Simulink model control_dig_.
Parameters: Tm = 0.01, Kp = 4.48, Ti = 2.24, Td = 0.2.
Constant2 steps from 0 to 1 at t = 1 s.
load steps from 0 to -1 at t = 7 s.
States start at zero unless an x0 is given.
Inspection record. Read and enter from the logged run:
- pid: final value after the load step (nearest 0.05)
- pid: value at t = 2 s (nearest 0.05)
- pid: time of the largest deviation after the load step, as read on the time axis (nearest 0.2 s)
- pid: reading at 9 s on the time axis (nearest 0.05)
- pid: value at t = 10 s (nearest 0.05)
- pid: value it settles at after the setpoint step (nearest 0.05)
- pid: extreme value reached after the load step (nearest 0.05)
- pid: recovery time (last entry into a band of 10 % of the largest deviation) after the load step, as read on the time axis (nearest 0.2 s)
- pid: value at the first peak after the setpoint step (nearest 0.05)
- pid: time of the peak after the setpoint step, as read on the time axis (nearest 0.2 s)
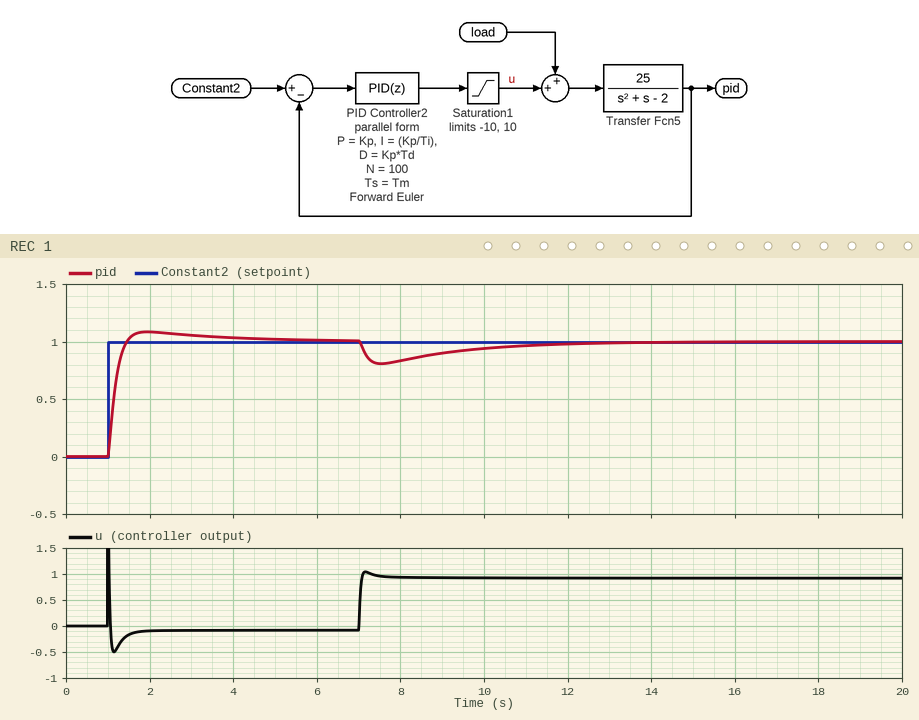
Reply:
1.00
1.10
7.6 s
0.90
0.95
1.00
0.80
12.2 s
1.10
2.0 s
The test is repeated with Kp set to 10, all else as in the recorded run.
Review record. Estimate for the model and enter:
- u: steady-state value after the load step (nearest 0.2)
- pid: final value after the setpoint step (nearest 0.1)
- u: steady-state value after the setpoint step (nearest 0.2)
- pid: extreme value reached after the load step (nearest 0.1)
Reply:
1.0
1.0
0.0
0.9
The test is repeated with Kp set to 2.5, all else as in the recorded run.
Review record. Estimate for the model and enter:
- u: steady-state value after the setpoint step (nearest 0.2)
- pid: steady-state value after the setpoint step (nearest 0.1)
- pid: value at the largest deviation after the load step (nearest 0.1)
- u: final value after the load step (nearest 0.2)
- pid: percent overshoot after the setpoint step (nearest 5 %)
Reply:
0.0
1.0
0.6
1.0
10 %
